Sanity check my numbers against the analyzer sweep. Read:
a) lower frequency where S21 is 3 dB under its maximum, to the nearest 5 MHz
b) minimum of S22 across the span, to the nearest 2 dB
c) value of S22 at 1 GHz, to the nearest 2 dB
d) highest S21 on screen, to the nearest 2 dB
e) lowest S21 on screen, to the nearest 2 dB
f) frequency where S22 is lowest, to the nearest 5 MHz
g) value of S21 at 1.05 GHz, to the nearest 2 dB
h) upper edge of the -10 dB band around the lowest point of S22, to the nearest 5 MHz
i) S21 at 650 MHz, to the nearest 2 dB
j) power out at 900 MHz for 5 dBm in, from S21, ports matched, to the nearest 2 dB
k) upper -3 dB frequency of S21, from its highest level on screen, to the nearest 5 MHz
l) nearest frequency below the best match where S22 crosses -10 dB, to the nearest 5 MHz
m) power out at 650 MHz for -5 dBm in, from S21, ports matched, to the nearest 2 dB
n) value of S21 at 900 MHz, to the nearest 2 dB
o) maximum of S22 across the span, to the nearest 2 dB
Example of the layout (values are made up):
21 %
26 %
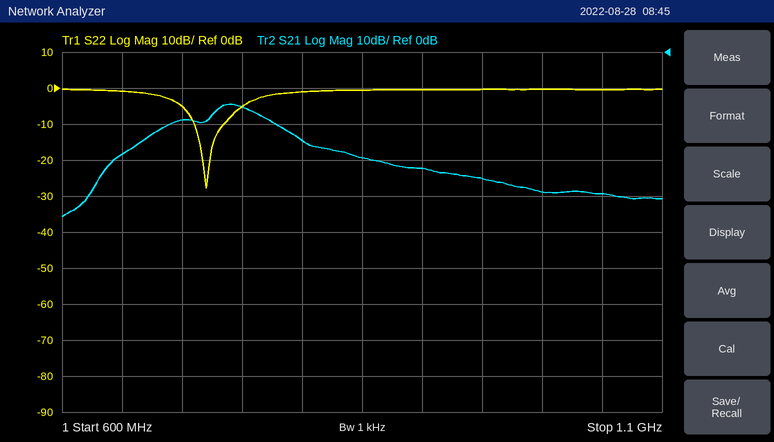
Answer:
725 MHz
-28 dB
0 dB
-14 dB
-46 dB
720 MHz
-40 dB
735 MHz
-28 dB
-28 dBm
765 MHz
710 MHz
-34 dBm
-32 dB
0 dB
